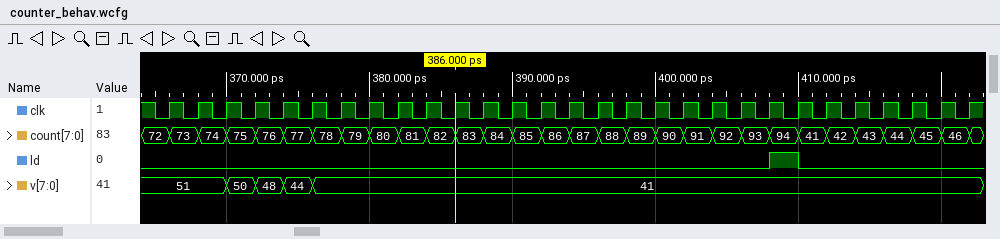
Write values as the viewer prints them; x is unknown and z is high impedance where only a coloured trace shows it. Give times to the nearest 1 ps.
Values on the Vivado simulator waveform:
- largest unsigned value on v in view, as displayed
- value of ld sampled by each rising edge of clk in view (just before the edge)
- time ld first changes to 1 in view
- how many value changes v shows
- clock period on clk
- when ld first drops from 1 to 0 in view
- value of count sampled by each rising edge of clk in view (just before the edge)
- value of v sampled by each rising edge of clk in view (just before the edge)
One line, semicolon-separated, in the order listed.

51; 0 0 0 0 0 0 0 0 0 0 0 0 0 0 0 0 0 0 0 0 0 0 1 0 0 0 0 0 0; 408 ps; 4; 2 ps; 410 ps; 72, 73, 74, 75, 76, 77, 78, 79, 80, 81, 82, 83, 84, 85, 86, 87, 88, 89, 90, 91, 92, 93, 94, 41, 42, 43, 44, 45, 46; 51, 51, 51, 50, 48, 44, 41, 41, 41, 41, 41, 41, 41, 41, 41, 41, 41, 41, 41, 41, 41, 41, 41, 41, 41, 41, 41, 41, 41
